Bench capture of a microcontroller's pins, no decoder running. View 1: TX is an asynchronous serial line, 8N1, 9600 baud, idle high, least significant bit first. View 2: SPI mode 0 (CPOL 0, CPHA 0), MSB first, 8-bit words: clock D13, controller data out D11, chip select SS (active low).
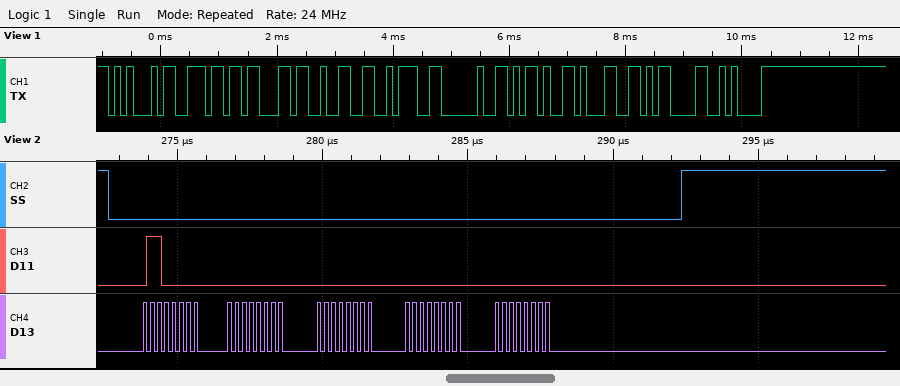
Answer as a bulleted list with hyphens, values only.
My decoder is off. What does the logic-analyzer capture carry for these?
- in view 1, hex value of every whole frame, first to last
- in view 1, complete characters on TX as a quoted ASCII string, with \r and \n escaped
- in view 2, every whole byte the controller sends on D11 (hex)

- 0x45 0x6E 0x63 0x32 0x3A 0x20 0x2D 0x31 0x0D 0x0A
- "Enc2: -1\r\n"
- 60 00 00 00 00
